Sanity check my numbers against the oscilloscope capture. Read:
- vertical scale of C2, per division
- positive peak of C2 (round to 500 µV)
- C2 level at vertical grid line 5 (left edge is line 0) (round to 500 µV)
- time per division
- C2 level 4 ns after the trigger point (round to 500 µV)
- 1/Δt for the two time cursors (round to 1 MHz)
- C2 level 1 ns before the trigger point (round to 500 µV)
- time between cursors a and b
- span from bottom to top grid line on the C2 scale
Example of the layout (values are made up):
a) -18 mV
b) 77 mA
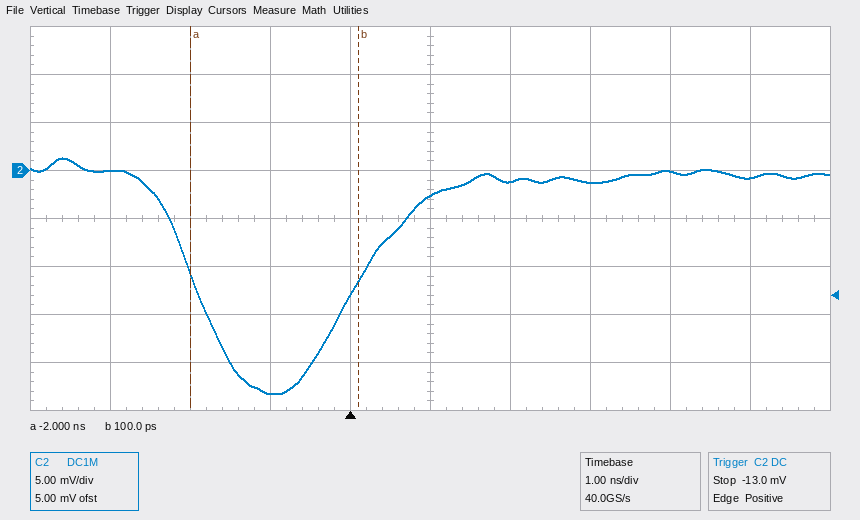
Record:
a) 5 mV
b) 1.5 mV
c) -2.5 mV
d) 1 ns
e) 0.0 mV
f) 476 MHz
g) -23.0 mV
h) 2.1 ns
i) 40 mV
